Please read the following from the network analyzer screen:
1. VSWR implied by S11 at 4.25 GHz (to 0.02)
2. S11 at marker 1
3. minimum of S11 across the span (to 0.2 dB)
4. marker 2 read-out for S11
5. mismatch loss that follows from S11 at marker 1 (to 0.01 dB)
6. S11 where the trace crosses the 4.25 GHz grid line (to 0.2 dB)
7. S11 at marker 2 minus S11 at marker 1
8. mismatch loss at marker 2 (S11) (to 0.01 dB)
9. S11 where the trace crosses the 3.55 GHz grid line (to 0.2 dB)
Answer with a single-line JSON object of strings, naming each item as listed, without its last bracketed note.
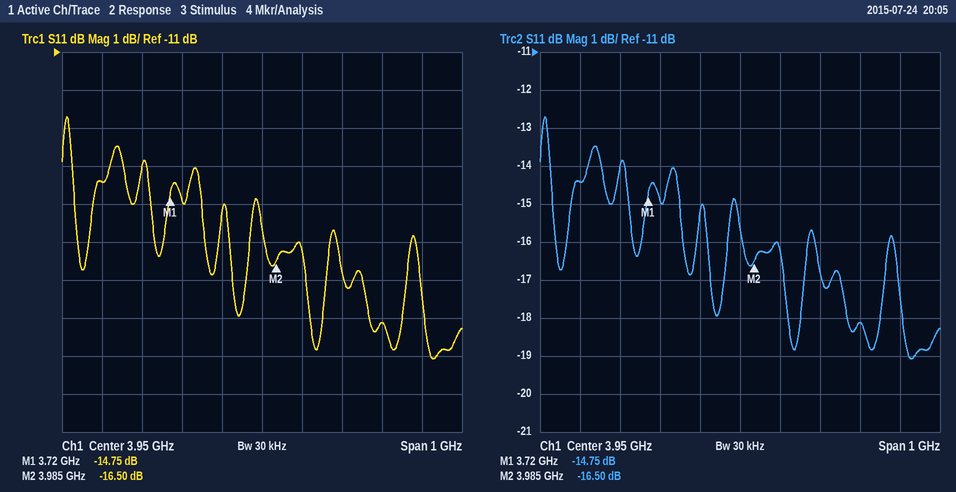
{"VSWR implied by S11 at 4.25 GHz": "1.28", "S11 at marker 1": "-14.75 dB", "minimum of S11 across the span": "-19.0 dB", "marker 2 read-out for S11": "-16.50 dB", "mismatch loss that follows from S11 at marker 1": "0.15 dB", "S11 where the trace crosses the 4.25 GHz grid line": "-18.2 dB", "S11 at marker 2 minus S11 at marker 1": "-1.75 dB", "mismatch loss at marker 2 (S11)": "0.10 dB", "S11 where the trace crosses the 3.55 GHz grid line": "-14.4 dB"}
